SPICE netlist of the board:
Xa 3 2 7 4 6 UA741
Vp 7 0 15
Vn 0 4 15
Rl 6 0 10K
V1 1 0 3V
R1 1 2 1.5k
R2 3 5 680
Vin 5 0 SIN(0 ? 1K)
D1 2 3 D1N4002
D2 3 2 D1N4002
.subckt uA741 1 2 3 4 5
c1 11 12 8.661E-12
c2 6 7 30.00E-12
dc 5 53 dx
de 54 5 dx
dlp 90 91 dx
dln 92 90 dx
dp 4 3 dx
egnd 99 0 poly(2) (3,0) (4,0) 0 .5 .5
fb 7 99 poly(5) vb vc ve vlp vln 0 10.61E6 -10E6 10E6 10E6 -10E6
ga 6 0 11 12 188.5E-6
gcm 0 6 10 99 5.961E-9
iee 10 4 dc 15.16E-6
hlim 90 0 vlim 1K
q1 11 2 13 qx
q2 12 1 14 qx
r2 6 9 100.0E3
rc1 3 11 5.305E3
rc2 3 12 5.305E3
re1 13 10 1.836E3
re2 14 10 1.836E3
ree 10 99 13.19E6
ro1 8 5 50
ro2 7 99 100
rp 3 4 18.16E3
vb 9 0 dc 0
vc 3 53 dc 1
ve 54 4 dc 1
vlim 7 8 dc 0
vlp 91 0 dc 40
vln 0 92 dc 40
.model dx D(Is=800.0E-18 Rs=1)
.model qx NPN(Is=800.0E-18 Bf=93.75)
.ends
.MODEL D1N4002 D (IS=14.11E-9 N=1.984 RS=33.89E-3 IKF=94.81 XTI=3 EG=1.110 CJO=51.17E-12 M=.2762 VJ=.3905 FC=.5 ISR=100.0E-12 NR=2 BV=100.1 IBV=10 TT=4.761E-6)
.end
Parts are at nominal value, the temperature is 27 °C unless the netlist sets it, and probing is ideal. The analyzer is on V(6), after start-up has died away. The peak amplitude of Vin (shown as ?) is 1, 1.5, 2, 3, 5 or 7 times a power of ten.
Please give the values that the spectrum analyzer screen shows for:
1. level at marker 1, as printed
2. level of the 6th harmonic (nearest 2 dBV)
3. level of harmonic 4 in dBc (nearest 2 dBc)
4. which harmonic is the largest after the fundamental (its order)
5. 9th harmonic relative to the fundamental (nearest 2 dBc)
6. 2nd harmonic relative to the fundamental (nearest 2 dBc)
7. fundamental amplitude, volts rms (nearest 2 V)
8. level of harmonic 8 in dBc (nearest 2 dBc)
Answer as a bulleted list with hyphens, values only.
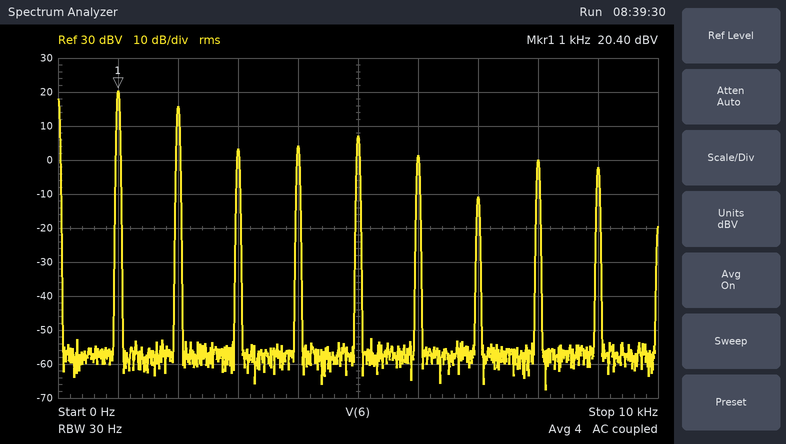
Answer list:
- 20.40 dBV
- 2 dBV
- -16 dBc
- 2
- -22 dBc
- -4 dBc
- 10 V
- -20 dBc
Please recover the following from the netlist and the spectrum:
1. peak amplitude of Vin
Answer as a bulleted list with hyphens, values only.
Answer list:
- 5 V
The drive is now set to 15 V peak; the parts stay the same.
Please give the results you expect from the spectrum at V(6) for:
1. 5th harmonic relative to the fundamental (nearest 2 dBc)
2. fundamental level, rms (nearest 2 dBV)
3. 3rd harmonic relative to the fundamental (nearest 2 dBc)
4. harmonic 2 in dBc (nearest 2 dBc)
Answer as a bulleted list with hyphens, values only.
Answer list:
- -20 dBc
- 22 dBV
- -12 dBc
- -14 dBc
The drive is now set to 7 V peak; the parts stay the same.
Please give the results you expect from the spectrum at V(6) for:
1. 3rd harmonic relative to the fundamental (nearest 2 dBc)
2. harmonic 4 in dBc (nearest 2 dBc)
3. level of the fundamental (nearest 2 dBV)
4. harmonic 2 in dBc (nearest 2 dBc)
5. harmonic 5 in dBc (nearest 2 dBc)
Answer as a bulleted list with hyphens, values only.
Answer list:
- -22 dBc
- -12 dBc
- 22 dBV
- -8 dBc
- -18 dBc
